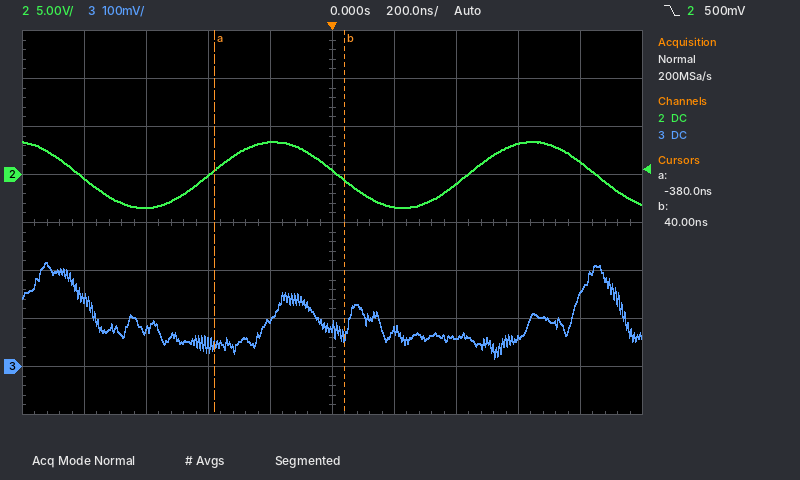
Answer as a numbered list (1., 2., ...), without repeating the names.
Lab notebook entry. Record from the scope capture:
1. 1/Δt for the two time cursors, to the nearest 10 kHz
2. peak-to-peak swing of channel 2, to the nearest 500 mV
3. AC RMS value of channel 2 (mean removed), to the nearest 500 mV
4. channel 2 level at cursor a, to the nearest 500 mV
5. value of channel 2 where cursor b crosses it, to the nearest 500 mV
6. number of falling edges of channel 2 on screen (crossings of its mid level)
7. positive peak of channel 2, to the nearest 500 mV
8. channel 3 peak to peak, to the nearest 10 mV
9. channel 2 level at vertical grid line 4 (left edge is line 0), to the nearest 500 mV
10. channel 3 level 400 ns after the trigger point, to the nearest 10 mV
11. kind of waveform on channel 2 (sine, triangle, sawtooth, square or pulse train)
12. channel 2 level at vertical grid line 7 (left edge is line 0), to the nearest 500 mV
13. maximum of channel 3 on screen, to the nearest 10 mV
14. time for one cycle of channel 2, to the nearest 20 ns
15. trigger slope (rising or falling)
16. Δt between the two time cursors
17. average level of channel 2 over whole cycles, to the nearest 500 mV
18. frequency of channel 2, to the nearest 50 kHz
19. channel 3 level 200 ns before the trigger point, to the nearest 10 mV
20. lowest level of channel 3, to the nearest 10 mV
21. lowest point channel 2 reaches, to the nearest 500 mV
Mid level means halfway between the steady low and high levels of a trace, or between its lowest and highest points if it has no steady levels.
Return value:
1. 2.38 MHz
2. 7.0 V
3. 2.5 V
4. 500 mV
5. -500 mV
6. 3
7. 3.5 V
8. 200 mV
9. 3.5 V
10. 60 mV
11. sine
12. -1.0 V
13. 220 mV
14. 840 ns
15. falling
16. 420 ns
17. 0.0 V
18. 1.20 MHz
19. 100 mV
20. 20 mV
21. -3.5 V
